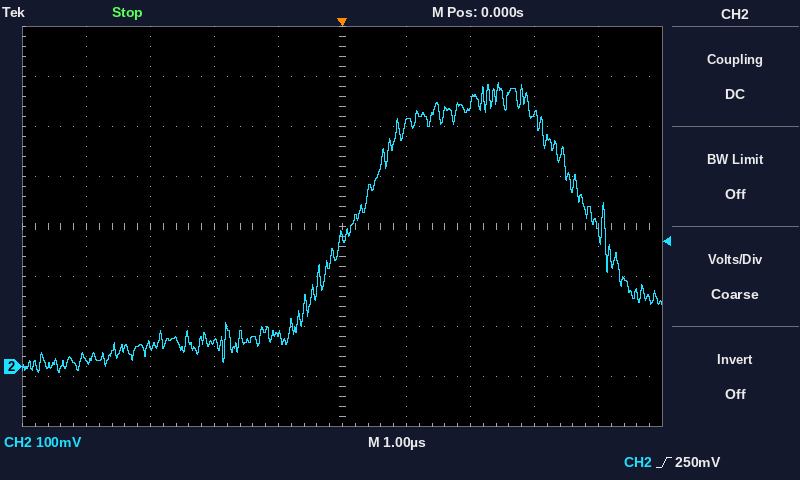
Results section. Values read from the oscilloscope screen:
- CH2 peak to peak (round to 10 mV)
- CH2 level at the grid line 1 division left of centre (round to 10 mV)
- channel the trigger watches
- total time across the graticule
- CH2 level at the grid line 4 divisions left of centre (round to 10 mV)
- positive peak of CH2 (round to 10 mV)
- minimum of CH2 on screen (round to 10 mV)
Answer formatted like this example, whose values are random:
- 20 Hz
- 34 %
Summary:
- 580 mV
- 60 mV
- CH2
- 10 µs
- 10 mV
- 570 mV
- -10 mV
